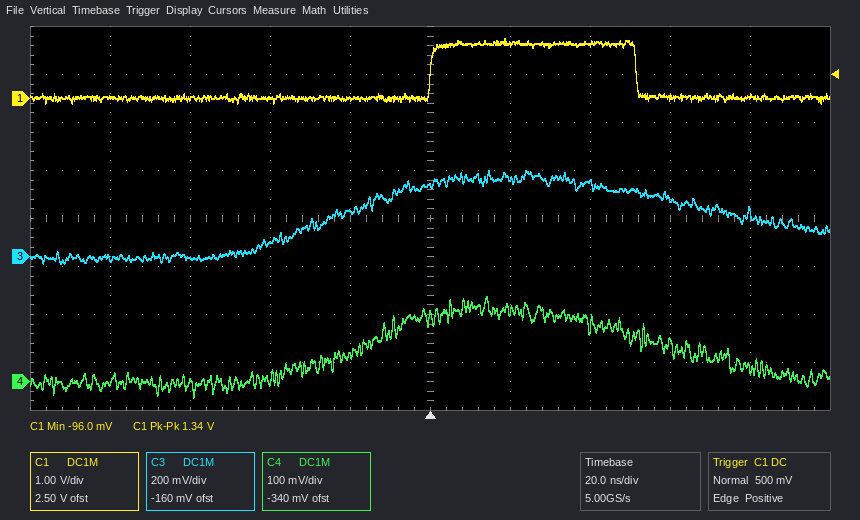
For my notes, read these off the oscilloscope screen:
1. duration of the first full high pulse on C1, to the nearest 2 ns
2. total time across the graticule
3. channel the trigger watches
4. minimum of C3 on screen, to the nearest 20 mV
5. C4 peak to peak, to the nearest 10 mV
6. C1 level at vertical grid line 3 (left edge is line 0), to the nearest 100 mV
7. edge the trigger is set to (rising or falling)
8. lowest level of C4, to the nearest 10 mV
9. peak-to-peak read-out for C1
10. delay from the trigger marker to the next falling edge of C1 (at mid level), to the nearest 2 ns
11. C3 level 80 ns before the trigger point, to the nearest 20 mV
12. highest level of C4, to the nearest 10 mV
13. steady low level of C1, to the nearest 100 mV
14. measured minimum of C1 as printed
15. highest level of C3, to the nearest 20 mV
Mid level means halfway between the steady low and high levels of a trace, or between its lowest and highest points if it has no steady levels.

52 ns
200 ns
C1
-20 mV
210 mV
0.0 V
rising
-30 mV
1.34 V
52 ns
0 mV
180 mV
0.0 V
-96.0 mV
360 mV
